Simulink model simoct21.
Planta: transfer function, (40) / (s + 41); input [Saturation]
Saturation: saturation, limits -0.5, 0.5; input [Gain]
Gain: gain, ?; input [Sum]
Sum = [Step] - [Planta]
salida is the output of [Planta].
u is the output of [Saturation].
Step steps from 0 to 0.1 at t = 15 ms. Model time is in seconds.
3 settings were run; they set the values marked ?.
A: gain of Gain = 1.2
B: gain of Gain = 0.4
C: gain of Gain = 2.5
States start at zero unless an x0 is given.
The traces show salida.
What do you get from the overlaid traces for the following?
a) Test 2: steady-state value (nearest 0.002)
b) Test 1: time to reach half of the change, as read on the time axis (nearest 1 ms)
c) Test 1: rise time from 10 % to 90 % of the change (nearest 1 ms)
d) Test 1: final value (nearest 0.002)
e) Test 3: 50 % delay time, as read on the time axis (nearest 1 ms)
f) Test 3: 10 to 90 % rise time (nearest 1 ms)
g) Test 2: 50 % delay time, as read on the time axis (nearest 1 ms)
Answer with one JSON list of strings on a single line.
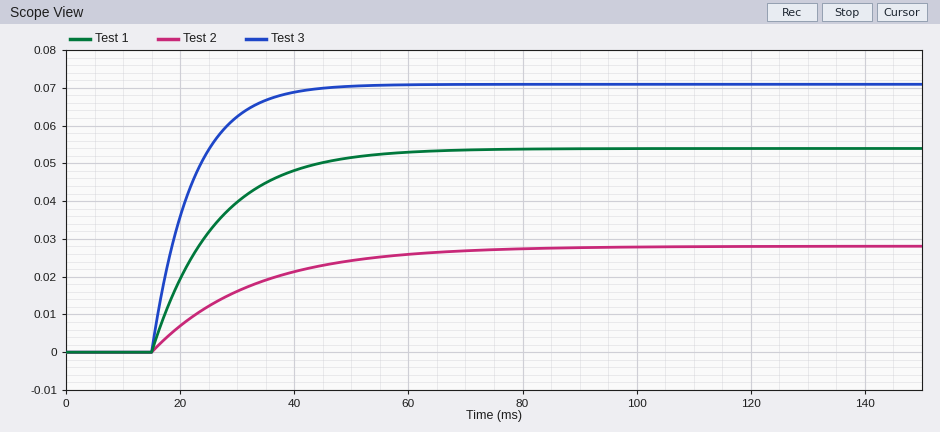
["0.028", "23 ms", "25 ms", "0.054", "20 ms", "16 ms", "27 ms"]
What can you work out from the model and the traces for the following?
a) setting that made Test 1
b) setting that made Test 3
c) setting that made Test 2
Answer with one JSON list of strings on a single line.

["A", "C", "B"]
